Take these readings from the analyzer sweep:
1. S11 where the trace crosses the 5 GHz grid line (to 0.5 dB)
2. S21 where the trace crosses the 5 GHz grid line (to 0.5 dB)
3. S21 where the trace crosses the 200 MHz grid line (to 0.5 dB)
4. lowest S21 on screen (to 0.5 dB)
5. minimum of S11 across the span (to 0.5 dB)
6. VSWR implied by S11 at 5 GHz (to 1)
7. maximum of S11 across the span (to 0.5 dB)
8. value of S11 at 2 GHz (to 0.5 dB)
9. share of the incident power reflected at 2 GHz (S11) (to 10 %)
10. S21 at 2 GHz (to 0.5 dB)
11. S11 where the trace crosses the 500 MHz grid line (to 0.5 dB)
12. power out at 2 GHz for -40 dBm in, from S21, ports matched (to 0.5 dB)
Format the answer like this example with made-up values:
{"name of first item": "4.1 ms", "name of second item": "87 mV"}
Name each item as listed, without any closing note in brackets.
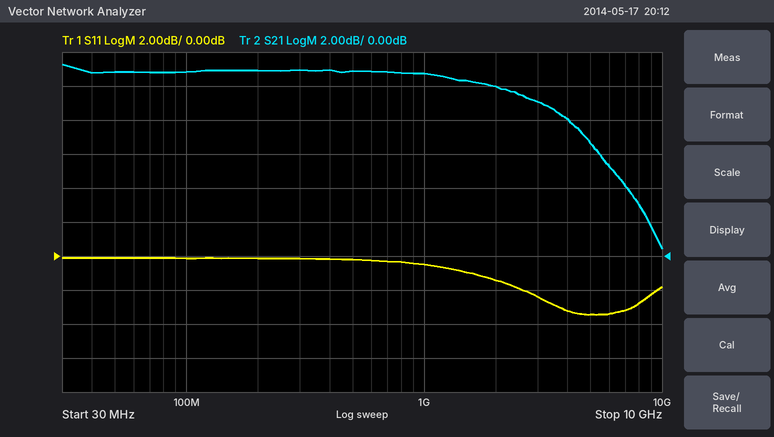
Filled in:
{"S11 where the trace crosses the 5 GHz grid line": "-3.5 dB", "S21 where the trace crosses the 5 GHz grid line": "6.5 dB", "S21 where the trace crosses the 200 MHz grid line": "11.0 dB", "lowest S21 on screen": "0.5 dB", "minimum of S11 across the span": "-3.5 dB", "VSWR implied by S11 at 5 GHz": "5", "maximum of S11 across the span": "0.0 dB", "value of S11 at 2 GHz": "-1.5 dB", "share of the incident power reflected at 2 GHz (S11)": "70 %", "S21 at 2 GHz": "10.0 dB", "S11 where the trace crosses the 500 MHz grid line": "0.0 dB", "power out at 2 GHz for -40 dBm in, from S21, ports matched": "-30.0 dBm"}
